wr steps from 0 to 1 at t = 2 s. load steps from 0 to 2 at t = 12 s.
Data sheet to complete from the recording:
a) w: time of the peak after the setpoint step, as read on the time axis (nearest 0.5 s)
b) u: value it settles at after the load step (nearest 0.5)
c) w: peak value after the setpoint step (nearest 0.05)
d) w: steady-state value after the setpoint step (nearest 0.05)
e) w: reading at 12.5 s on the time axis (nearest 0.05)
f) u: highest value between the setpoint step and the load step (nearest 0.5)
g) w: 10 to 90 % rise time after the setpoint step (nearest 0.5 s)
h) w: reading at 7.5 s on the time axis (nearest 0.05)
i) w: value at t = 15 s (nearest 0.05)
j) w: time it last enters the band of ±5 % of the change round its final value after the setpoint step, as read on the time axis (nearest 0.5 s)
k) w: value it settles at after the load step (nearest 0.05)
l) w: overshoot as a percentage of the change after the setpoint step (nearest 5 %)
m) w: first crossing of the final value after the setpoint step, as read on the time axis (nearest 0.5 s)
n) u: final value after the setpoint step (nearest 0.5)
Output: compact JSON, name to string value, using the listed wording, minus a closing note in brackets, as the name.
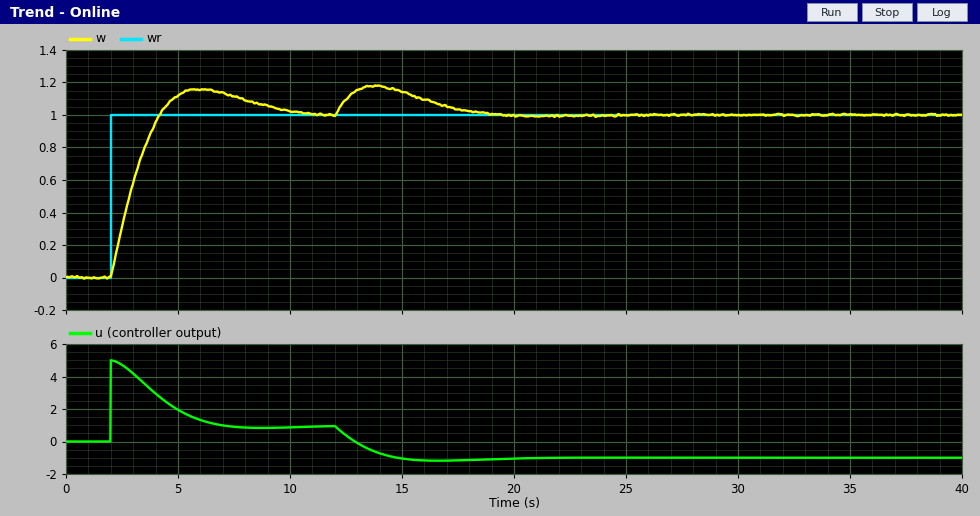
{"w: time of the peak after the setpoint step, as read on the time axis": "6.0 s", "u: value it settles at after the load step": "-1.0", "w: peak value after the setpoint step": "1.15", "w: steady-state value after the setpoint step": "1.00", "w: reading at 12.5 s on the time axis": "1.10", "u: highest value between the setpoint step and the load step": "5.0", "w: 10 to 90 % rise time after the setpoint step": "1.5 s", "w: reading at 7.5 s on the time axis": "1.10", "w: value at t = 15 s": "1.15", "w: time it last enters the band of ±5 % of the change round its final value after the setpoint step, as read on the time axis": "9.0 s", "w: value it settles at after the load step": "1.00", "w: overshoot as a percentage of the change after the setpoint step": "15 %", "w: first crossing of the final value after the setpoint step, as read on the time axis": "4.0 s", "u: final value after the setpoint step": "1.0"}
